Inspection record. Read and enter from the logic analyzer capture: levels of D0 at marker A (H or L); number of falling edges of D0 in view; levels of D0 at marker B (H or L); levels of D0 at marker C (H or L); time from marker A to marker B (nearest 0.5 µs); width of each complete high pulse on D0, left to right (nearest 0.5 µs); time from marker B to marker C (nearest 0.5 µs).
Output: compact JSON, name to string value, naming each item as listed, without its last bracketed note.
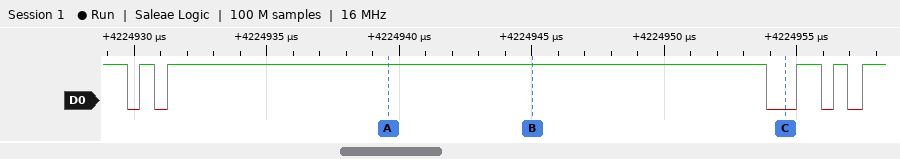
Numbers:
{"levels of D0 at marker A": "D0=H", "number of falling edges of D0 in view": "5", "levels of D0 at marker B": "D0=H", "levels of D0 at marker C": "D0=L", "time from marker A to marker B": "5.5 µs", "width of each complete high pulse on D0, left to right": "0.5 µs, 22.5 µs, 1 µs, 0.5 µs", "time from marker B to marker C": "9.5 µs"}
